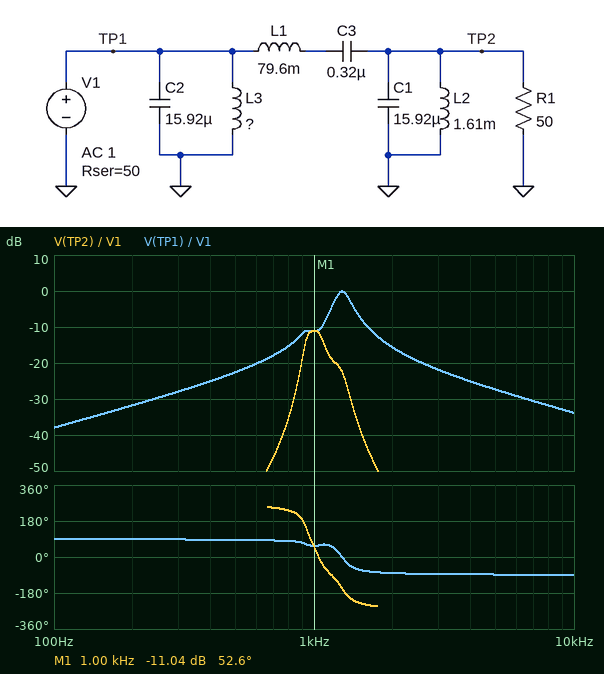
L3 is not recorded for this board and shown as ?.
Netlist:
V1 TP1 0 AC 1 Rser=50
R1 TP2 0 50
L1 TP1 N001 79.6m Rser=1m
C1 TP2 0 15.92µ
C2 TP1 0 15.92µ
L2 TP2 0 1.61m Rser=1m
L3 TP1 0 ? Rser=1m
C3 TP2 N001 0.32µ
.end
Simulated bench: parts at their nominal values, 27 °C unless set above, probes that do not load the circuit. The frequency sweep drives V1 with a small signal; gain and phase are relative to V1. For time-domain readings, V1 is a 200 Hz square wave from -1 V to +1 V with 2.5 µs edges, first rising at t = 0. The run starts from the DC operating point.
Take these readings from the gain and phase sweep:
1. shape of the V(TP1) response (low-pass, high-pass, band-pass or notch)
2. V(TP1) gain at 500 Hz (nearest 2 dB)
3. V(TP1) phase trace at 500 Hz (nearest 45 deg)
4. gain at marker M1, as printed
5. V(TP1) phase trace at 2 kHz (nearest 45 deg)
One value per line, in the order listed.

band-pass
-22 dB
90 deg
-11.04 dB
-90 deg
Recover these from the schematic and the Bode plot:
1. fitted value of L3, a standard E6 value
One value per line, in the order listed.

1 mH
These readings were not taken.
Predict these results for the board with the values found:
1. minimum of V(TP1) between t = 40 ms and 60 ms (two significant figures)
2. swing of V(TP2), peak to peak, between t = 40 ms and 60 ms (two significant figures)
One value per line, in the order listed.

-260 mV
150 mV
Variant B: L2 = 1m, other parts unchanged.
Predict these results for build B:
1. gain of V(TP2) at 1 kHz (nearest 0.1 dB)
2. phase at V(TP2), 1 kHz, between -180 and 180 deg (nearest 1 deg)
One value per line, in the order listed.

-16.6 dB
70 deg
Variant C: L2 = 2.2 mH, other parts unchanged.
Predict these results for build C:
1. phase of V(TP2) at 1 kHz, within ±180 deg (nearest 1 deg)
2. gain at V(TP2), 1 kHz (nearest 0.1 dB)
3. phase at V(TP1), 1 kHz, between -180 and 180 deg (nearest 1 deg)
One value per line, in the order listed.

32 deg
-7.8 dB
35 deg
